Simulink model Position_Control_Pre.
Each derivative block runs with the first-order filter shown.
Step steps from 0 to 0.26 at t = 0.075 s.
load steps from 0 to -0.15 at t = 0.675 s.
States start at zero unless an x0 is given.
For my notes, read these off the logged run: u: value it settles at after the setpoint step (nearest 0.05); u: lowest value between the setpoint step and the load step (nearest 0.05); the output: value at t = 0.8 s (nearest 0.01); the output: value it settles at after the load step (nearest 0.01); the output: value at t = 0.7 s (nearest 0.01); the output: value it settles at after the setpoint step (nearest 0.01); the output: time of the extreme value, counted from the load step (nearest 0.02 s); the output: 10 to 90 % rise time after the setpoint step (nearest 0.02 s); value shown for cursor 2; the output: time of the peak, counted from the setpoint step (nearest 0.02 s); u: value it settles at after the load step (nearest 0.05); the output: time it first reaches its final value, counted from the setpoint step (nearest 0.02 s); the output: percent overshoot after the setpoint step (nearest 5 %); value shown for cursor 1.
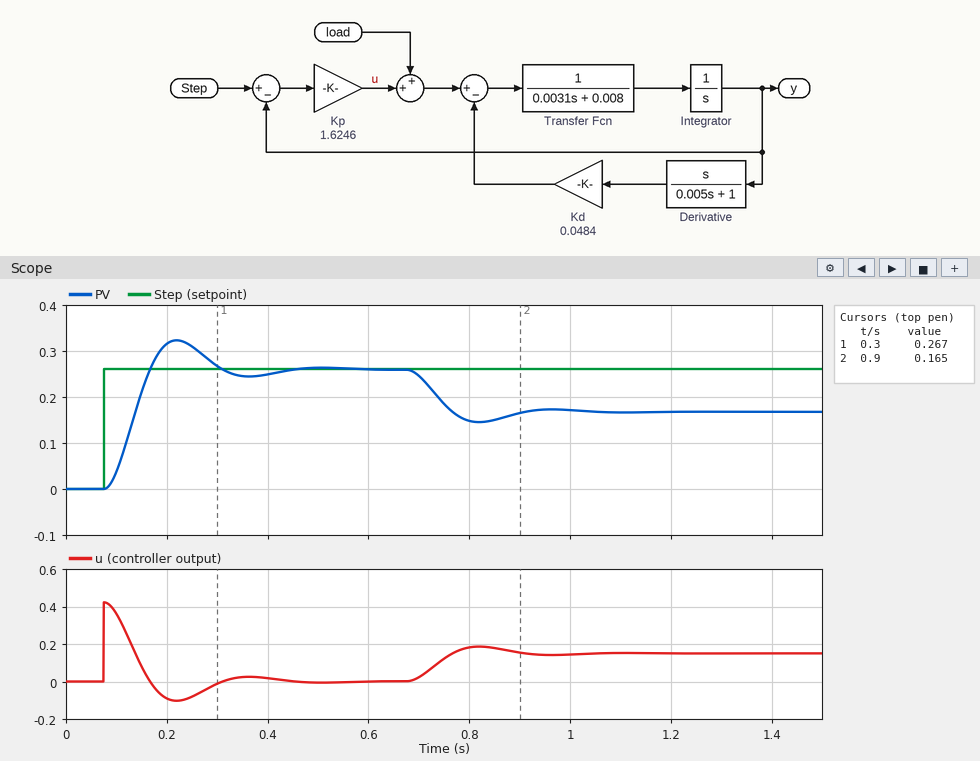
0.00
-0.10
0.15
0.17
0.25
0.26
0.14 s
0.06 s
0.165
0.14 s
0.15
0.10 s
25 %
0.267
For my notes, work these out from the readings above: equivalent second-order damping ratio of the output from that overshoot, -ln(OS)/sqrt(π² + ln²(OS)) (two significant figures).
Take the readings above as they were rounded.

0.40
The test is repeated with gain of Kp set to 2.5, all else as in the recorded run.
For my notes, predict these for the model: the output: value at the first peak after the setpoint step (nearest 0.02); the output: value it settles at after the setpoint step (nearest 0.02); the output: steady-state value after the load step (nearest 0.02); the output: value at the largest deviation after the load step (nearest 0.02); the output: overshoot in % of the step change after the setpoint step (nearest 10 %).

0.34
0.26
0.20
0.18
30 %
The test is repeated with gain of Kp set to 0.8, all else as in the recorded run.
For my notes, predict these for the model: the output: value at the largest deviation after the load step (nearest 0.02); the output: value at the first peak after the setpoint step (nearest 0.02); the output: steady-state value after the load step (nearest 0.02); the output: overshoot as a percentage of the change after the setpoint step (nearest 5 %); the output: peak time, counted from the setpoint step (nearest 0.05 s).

0.06
0.28
0.08
10 %
0.25 s
